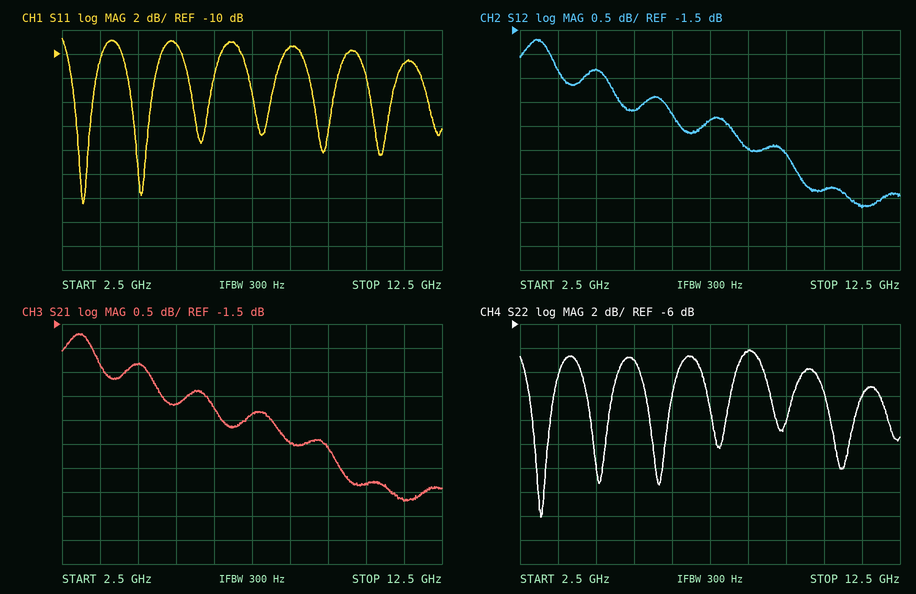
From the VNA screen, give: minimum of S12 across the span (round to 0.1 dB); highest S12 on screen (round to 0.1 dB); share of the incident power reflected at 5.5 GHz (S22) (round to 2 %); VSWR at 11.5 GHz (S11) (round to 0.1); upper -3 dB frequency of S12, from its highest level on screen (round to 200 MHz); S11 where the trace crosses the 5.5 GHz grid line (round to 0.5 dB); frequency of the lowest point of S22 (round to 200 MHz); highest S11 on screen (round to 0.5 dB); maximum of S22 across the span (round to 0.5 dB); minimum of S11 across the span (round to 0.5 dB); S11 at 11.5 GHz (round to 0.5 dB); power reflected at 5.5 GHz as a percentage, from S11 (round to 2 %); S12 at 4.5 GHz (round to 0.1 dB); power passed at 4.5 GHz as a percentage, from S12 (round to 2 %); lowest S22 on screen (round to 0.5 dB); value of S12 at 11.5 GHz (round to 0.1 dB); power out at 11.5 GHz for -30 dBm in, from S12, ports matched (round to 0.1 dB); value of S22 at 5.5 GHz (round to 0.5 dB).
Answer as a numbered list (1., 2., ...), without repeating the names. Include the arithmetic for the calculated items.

1. -5.2 dB
2. -1.7 dB
3. 10^(-9/10) ≈ 12.6 %, so 12 % to the nearest 2 %
4. |Γ| = 10^(-11/20) = 0.2818; VSWR = (1 + 0.2818)/(1 − 0.2818) ≈ 1.8
5. 10.0 GHz
6. -9.0 dB
7. 3.0 GHz
8. -8.5 dB
9. -8.0 dB
10. -22.5 dB
11. -11.0 dB
12. 10^(-9/10) ≈ 12.6 %, so 12 % to the nearest 2 %
13. -2.3 dB
14. 10^(-2.3/10) ≈ 58.9 %, so 58 % to the nearest 2 %
15. -22.0 dB
16. -5.2 dB
17. -30 dBm + (-5.2 dB) = -35.2 dBm
18. -9.0 dB
